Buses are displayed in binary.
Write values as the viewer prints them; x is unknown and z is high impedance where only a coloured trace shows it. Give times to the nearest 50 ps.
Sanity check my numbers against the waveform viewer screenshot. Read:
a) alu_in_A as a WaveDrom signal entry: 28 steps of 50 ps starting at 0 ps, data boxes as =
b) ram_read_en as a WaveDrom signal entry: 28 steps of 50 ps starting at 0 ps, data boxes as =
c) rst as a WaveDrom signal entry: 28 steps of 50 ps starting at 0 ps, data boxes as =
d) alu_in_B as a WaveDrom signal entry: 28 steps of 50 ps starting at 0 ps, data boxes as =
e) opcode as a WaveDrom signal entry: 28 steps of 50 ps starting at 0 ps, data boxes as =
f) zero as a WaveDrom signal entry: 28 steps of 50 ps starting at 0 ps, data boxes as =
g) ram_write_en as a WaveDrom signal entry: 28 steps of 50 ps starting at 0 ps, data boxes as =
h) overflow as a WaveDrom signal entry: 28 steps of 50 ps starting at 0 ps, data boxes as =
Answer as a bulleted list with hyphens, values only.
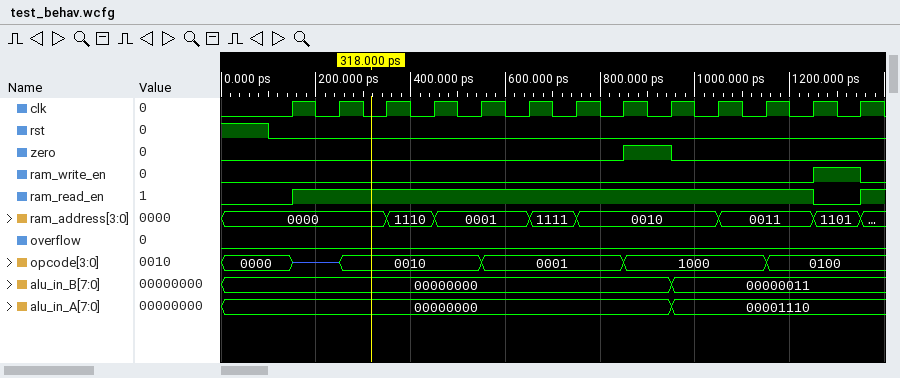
- {name: 'alu_in_A', wave: '=..................=........', data: '00000000 00001110'}
- {name: 'ram_read_en', wave: '0..1.....................0.1'}
- {name: 'rst', wave: '1.0.........................'}
- {name: 'alu_in_B', wave: '=..................=........', data: '00000000 00000011'}
- {name: 'opcode', wave: '=..z.=.....=.....=.....=....', data: '0000 0010 0001 1000 0100'}
- {name: 'zero', wave: '0................1.0........'}
- {name: 'ram_write_en', wave: '0........................1.0'}
- {name: 'overflow', wave: '0...........................'}
